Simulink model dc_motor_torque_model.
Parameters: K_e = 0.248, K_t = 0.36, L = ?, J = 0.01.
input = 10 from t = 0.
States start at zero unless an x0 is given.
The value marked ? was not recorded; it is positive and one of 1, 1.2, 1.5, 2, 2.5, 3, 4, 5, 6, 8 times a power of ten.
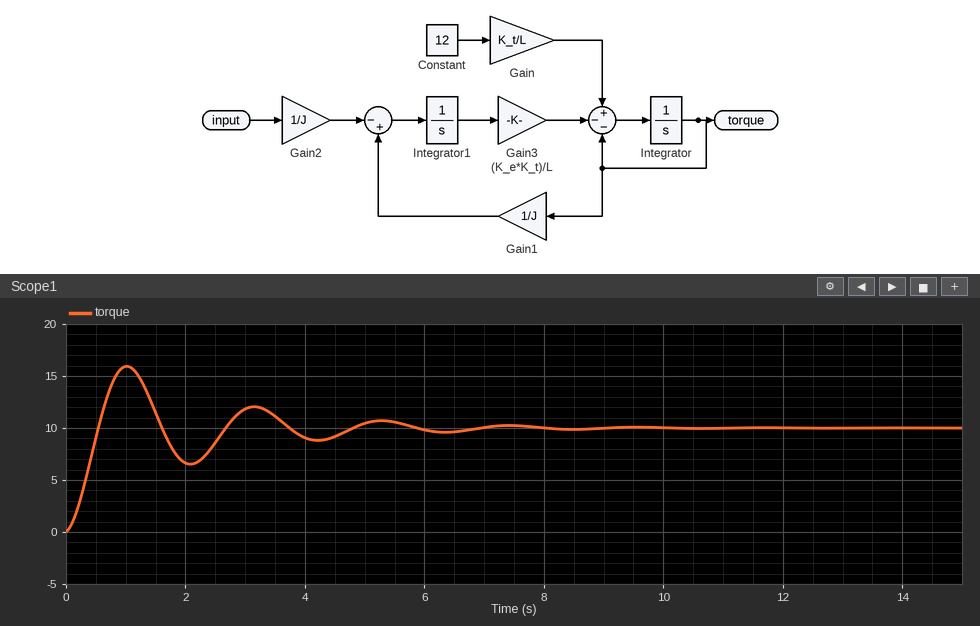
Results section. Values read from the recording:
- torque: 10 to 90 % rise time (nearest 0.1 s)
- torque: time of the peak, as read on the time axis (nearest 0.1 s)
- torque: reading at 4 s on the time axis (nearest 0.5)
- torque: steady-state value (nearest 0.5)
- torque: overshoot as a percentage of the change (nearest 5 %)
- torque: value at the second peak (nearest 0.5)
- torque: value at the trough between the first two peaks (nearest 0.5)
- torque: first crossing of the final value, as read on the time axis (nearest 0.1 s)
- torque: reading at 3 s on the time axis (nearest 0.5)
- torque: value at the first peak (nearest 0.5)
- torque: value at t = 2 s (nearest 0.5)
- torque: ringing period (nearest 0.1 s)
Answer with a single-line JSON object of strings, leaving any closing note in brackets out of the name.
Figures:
{"torque: 10 to 90 % rise time": "0.4 s", "torque: time of the peak, as read on the time axis": "1.0 s", "torque: reading at 4 s on the time axis": "9.0", "torque: steady-state value": "10.0", "torque: overshoot as a percentage of the change": "60 %", "torque: value at the second peak": "12.0", "torque: value at the trough between the first two peaks": "6.5", "torque: first crossing of the final value, as read on the time axis": "0.5 s", "torque: reading at 3 s on the time axis": "12.0", "torque: value at the first peak": "16.0", "torque: value at t = 2 s": "6.5", "torque: ringing period": "2.1 s"}
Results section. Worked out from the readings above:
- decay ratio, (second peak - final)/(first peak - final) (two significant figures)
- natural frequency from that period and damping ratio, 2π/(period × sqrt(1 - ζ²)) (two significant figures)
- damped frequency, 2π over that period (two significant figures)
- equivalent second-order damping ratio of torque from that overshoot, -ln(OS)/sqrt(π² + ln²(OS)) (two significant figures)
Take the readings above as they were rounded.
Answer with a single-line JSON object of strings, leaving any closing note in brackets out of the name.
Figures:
{"decay ratio, (second peak - final)/(first peak - final)": "0.33", "natural frequency from that period and damping ratio, 2π/(period × sqrt(1 - ζ²))": "3.0 rad/s", "damped frequency, 2π over that period": "3.0 rad/s", "equivalent second-order damping ratio of torque from that overshoot, -ln(OS)/sqrt(π² + ln²(OS))": "0.16"}
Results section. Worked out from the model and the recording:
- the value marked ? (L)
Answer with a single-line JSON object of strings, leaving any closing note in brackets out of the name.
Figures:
{"the value marked ?": "1"}
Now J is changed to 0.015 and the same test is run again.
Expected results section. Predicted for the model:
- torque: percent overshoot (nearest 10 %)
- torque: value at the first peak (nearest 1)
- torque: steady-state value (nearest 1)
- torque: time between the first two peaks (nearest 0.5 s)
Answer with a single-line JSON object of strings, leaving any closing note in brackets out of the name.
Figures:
{"torque: percent overshoot": "50 %", "torque: value at the first peak": "15", "torque: steady-state value": "10", "torque: time between the first two peaks": "2.5 s"}
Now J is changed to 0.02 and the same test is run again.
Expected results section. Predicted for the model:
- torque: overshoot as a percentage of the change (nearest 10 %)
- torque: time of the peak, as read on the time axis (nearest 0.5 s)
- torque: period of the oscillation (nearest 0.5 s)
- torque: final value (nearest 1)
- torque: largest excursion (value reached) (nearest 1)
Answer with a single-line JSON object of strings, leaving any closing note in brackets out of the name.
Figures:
{"torque: overshoot as a percentage of the change": "50 %", "torque: time of the peak, as read on the time axis": "1.5 s", "torque: period of the oscillation": "3.0 s", "torque: final value": "10", "torque: largest excursion (value reached)": "15"}
